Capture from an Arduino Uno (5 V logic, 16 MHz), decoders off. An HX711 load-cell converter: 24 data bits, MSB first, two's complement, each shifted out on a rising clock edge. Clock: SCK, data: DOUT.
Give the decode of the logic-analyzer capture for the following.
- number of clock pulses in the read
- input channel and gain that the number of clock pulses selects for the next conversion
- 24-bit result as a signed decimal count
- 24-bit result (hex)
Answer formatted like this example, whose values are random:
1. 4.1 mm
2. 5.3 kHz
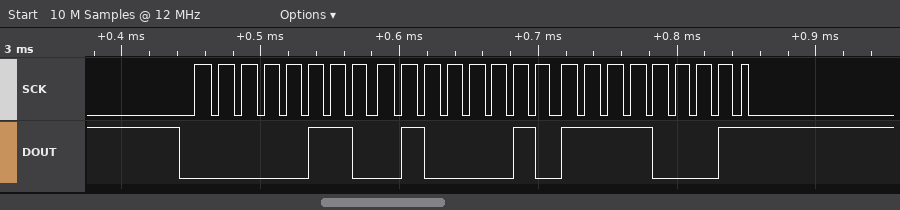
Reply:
1. 25
2. channel A, gain 128
3. 410353
4. 0x0642F1
